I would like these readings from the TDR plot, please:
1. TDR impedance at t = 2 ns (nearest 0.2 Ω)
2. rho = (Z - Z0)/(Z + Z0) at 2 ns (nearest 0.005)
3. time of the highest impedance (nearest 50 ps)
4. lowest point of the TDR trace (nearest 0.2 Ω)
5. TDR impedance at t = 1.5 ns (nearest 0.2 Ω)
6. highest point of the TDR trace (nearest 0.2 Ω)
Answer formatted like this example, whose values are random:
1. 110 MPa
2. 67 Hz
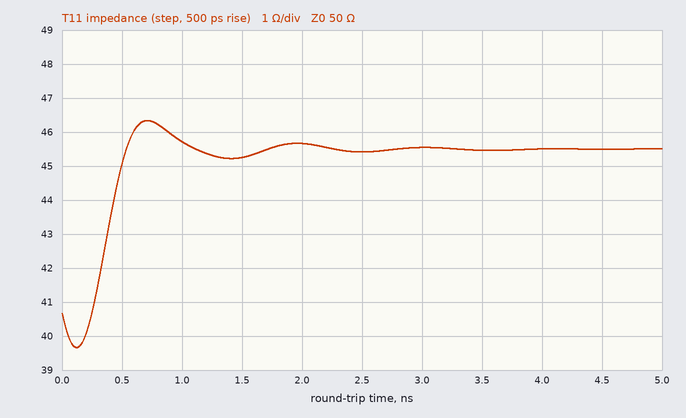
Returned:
1. 45.6 Ω
2. -0.045
3. 700 ps
4. 39.6 Ω
5. 45.2 Ω
6. 46.4 Ω
